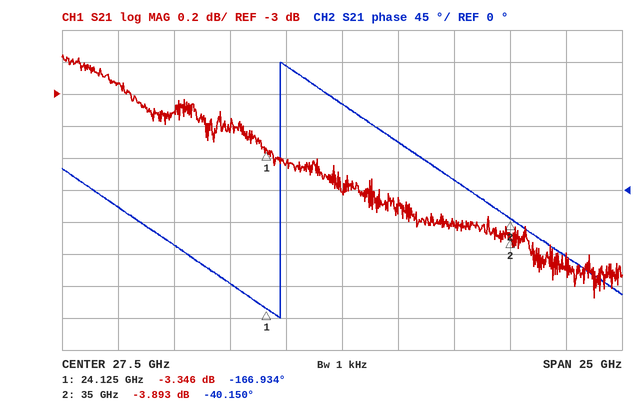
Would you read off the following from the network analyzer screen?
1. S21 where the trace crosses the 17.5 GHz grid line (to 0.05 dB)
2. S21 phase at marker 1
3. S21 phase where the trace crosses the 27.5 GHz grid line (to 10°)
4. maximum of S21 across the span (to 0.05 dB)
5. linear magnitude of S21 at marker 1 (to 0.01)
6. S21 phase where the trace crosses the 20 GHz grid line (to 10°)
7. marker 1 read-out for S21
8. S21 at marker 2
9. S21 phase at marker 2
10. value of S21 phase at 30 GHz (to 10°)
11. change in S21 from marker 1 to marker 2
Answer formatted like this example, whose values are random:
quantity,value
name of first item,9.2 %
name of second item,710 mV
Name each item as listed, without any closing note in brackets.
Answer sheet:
quantity,value
S21 where the trace crosses the 17.5 GHz grid line,-2.95 dB
S21 phase at marker 1,-166.934°
S21 phase where the trace crosses the 27.5 GHz grid line,120°
maximum of S21 across the span,-2.75 dB
linear magnitude of S21 at marker 1,0.68
S21 phase where the trace crosses the 20 GHz grid line,-80°
marker 1 read-out for S21,-3.346 dB
S21 at marker 2,-3.893 dB
S21 phase at marker 2,-40.150°
value of S21 phase at 30 GHz,70°
change in S21 from marker 1 to marker 2,-0.547 dB
